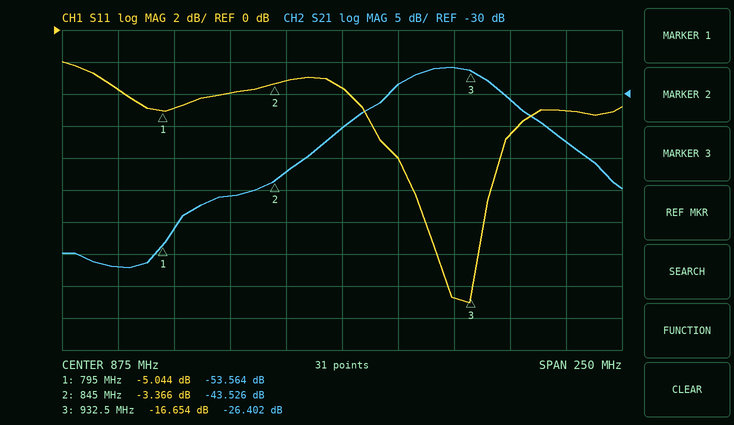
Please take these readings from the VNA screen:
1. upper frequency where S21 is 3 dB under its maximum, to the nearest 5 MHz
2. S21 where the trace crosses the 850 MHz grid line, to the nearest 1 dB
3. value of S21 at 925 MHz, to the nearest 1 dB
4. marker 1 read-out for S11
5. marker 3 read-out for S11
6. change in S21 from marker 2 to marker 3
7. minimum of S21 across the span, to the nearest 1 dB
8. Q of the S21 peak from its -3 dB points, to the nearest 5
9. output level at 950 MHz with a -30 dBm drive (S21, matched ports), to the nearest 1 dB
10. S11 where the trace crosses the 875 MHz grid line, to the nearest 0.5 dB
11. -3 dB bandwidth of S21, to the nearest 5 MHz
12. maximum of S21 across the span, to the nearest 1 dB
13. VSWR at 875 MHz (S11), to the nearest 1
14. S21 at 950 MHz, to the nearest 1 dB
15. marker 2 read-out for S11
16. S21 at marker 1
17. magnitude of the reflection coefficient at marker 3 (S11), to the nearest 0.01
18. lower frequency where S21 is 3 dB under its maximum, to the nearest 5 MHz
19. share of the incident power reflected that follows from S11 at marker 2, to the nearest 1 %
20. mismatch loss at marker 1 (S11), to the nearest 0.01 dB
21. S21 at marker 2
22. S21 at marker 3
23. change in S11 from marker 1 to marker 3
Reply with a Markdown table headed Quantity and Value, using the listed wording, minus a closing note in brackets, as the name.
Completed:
| Quantity | Value |
|---|---|
| upper frequency where S21 is 3 dB under its maximum, to the nearest 5 MHz | 945 MHz |
| S21 where the trace crosses the 850 MHz grid line, to the nearest 1 dB | -42 dB |
| value of S21 at 925 MHz, to the nearest 1 dB | -26 dB |
| marker 1 read-out for S11 | -5.044 dB |
| marker 3 read-out for S11 | -16.654 dB |
| change in S21 from marker 2 to marker 3 | 17.124 dB |
| minimum of S21 across the span, to the nearest 1 dB | -57 dB |
| Q of the S21 peak from its -3 dB points, to the nearest 5 | 20 |
| output level at 950 MHz with a -30 dBm drive (S21, matched ports), to the nearest 1 dB | -61 dBm |
| S11 where the trace crosses the 875 MHz grid line, to the nearest 0.5 dB | -3.5 dB |
| -3 dB bandwidth of S21, to the nearest 5 MHz | 45 MHz |
| maximum of S21 across the span, to the nearest 1 dB | -26 dB |
| VSWR at 875 MHz (S11), to the nearest 1 | 5 |
| S21 at 950 MHz, to the nearest 1 dB | -31 dB |
| marker 2 read-out for S11 | -3.366 dB |
| S21 at marker 1 | -53.564 dB |
| magnitude of the reflection coefficient at marker 3 (S11), to the nearest 0.01 | 0.15 |
| lower frequency where S21 is 3 dB under its maximum, to the nearest 5 MHz | 900 MHz |
| share of the incident power reflected that follows from S11 at marker 2, to the nearest 1 % | 46 % |
| mismatch loss at marker 1 (S11), to the nearest 0.01 dB | 1.63 dB |
| S21 at marker 2 | -43.526 dB |
| S21 at marker 3 | -26.402 dB |
| change in S11 from marker 1 to marker 3 | -11.610 dB |
